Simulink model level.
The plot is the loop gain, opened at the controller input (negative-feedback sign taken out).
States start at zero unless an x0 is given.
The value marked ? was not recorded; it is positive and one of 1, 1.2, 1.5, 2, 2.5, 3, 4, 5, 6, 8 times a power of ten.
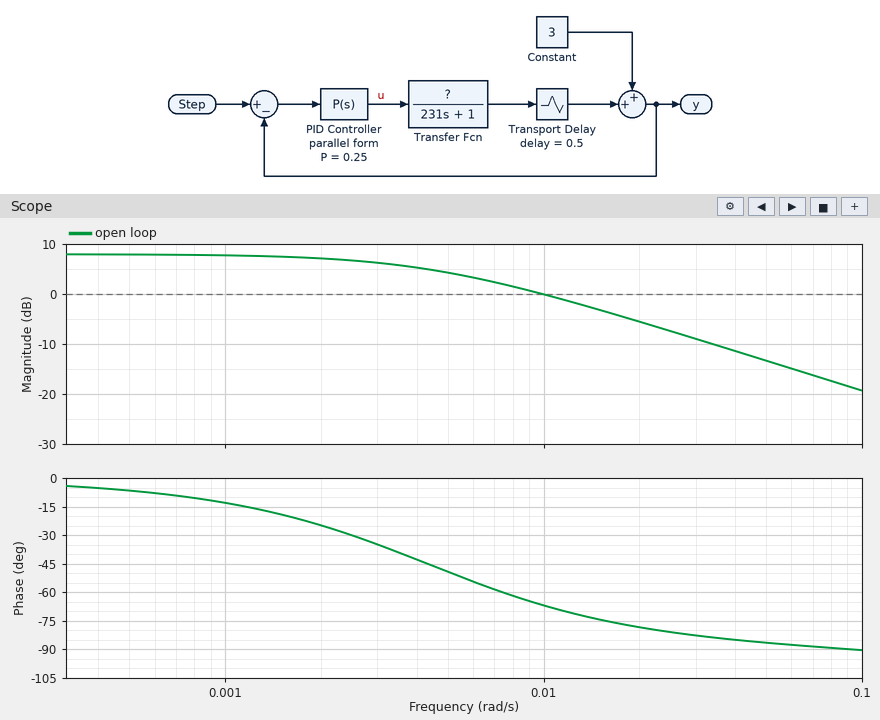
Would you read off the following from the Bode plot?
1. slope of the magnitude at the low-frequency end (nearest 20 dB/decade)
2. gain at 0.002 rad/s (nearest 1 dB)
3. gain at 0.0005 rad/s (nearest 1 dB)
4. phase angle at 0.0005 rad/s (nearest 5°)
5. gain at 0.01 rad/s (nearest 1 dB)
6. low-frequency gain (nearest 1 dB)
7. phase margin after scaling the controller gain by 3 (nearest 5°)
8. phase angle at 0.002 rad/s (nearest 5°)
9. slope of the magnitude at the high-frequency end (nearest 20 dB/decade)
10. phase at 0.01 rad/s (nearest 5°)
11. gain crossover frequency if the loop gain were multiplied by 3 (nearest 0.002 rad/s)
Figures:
0 dB/decade
7 dB
8 dB
-5°
0 dB
8 dB
95°
-25°
-20 dB/decade
-65°
0.032 rad/s
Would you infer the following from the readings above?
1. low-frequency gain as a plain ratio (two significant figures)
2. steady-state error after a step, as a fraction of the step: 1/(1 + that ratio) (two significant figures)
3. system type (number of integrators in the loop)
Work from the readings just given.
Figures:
2.5
0.29
0
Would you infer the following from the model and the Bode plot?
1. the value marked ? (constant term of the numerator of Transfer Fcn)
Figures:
10
